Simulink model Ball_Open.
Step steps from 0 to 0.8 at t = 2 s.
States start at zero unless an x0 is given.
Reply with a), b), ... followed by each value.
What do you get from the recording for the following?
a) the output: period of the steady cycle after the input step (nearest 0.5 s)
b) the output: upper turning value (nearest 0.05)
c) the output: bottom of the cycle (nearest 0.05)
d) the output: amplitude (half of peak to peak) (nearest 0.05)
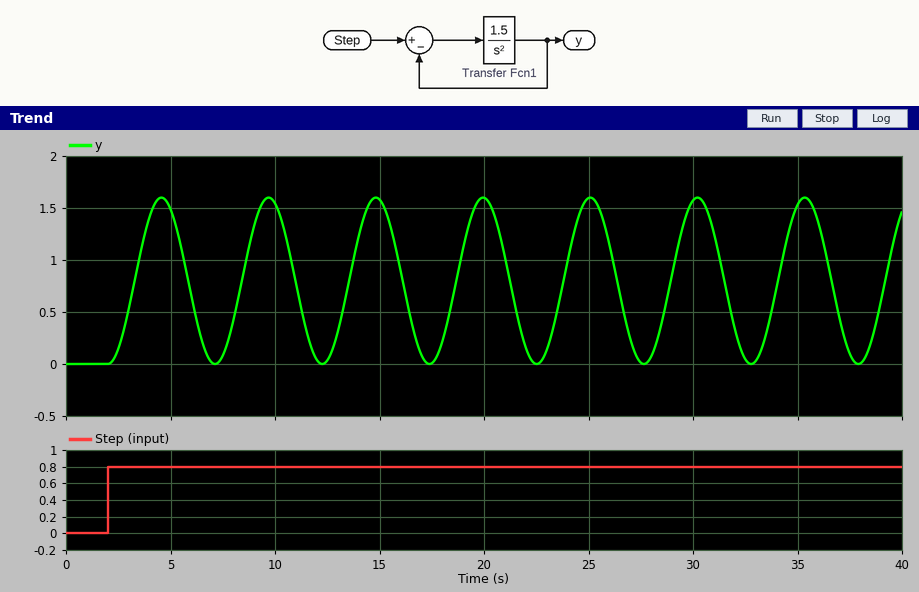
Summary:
a) 5.0 s
b) 1.60
c) 0.00
d) 0.80
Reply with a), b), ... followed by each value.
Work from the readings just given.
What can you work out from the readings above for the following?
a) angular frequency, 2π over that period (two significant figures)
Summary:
a) 1.3 rad/s
